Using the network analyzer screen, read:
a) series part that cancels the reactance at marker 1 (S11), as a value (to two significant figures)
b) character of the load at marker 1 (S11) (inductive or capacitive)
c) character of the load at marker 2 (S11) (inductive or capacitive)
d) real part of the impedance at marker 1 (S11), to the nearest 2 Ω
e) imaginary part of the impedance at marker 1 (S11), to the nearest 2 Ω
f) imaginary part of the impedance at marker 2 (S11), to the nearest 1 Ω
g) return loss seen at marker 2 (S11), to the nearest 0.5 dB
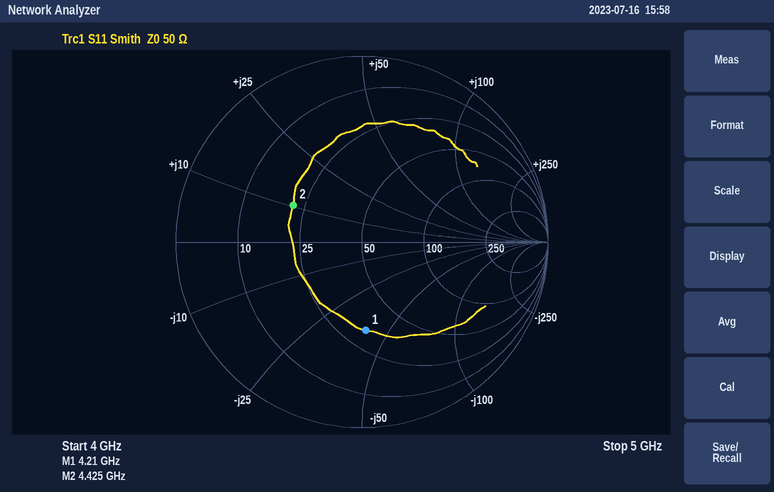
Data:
1.5 nH
capacitive
inductive
32 Ω
-40 Ω
+10 Ω
7.5 dB
